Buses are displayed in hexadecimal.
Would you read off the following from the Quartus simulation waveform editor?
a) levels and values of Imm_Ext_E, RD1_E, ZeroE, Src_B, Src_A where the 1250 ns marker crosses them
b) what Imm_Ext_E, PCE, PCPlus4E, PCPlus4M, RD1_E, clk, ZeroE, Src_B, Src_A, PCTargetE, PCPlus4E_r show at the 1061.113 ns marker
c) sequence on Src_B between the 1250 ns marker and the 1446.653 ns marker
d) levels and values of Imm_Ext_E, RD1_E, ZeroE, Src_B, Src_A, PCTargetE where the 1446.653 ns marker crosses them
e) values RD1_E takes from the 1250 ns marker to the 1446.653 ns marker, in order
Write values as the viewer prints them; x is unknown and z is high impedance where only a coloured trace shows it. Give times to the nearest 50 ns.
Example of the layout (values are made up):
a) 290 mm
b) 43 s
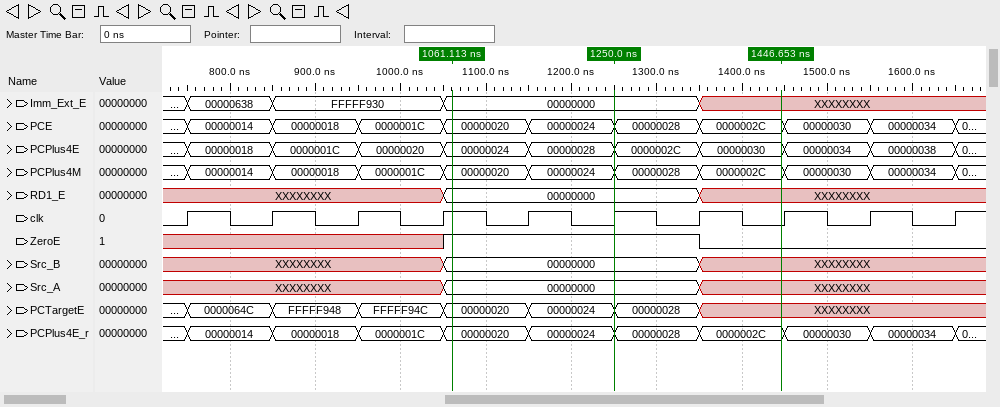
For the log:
a) Imm_Ext_E=00000000, RD1_E=00000000, ZeroE=1, Src_B=00000000, Src_A=00000000
b) Imm_Ext_E=00000000, PCE=00000020, PCPlus4E=00000024, PCPlus4M=00000020, RD1_E=00000000, clk=1, ZeroE=1, Src_B=00000000, Src_A=00000000, PCTargetE=00000020, PCPlus4E_r=00000020
c) 00000000, XXXXXXXX
d) Imm_Ext_E=XXXXXXXX, RD1_E=XXXXXXXX, ZeroE=0, Src_B=XXXXXXXX, Src_A=XXXXXXXX, PCTargetE=XXXXXXXX
e) 00000000, XXXXXXXX
